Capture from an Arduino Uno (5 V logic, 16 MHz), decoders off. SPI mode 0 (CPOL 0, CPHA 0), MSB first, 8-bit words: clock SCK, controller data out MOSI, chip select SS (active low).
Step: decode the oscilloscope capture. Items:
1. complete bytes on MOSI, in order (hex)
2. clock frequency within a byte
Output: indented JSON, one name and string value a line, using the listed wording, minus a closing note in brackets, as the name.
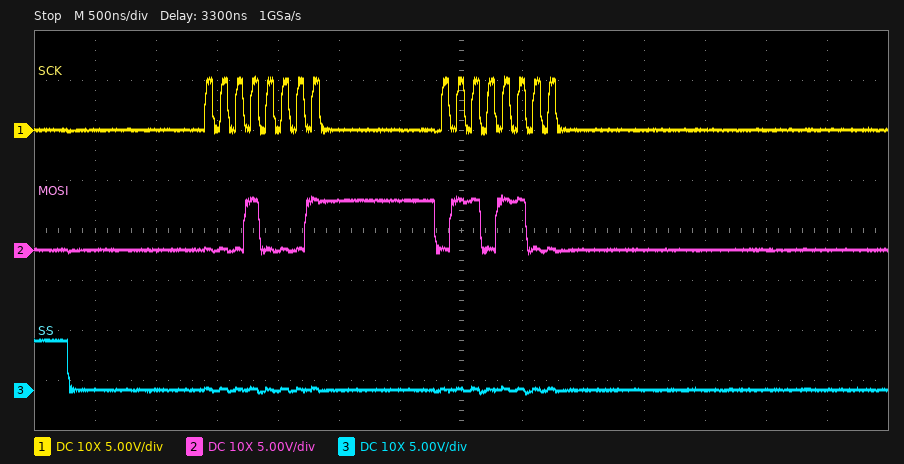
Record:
{
  "complete bytes on MOSI, in order": "11 6C",
  "clock frequency within a byte": "8 MHz"
}
